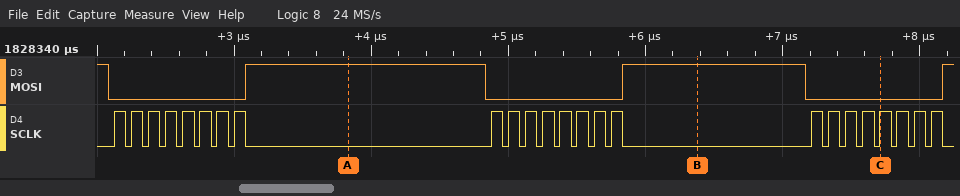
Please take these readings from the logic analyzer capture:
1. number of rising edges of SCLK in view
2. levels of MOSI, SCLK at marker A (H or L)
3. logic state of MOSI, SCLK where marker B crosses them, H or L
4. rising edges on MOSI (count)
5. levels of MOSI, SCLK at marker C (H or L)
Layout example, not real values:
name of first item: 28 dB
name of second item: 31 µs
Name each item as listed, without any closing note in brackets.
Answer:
number of rising edges of SCLK in view: 24
levels of MOSI, SCLK at marker A: MOSI=H, SCLK=L
logic state of MOSI, SCLK where marker B crosses them, H or L: MOSI=H, SCLK=L
rising edges on MOSI: 3
levels of MOSI, SCLK at marker C: MOSI=L, SCLK=H
